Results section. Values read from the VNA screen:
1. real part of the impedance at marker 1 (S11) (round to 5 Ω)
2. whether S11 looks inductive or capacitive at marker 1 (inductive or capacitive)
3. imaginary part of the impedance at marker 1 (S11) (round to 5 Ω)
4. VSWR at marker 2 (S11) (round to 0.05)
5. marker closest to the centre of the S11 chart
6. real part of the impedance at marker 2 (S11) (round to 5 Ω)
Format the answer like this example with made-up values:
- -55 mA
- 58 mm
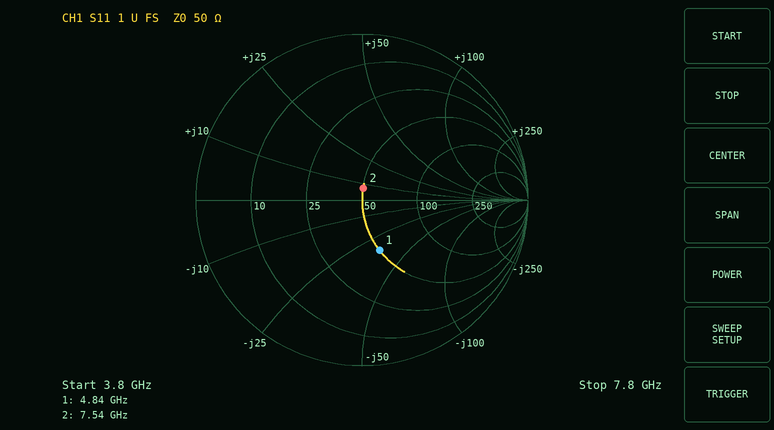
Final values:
- 50 Ω
- capacitive
- -35 Ω
- 1.15
- marker 2
- 50 Ω
